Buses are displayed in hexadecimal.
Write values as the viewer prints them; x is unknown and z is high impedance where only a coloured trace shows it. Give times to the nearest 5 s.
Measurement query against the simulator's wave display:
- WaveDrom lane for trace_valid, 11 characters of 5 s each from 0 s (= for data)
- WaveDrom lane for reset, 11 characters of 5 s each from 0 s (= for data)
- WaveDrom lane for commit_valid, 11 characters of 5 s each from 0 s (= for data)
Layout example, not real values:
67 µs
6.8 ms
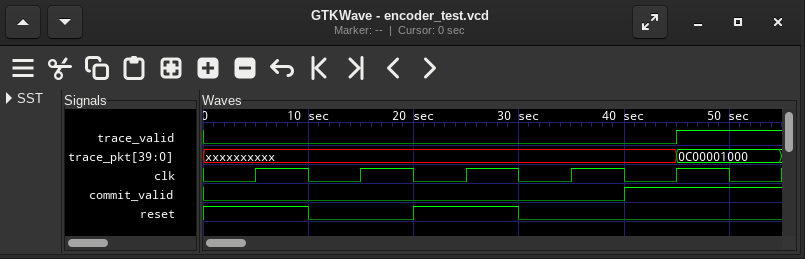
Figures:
{name: 'trace_valid', wave: '0........1.'}
{name: 'reset', wave: '1.0.1.0....'}
{name: 'commit_valid', wave: '0.......1..'}
